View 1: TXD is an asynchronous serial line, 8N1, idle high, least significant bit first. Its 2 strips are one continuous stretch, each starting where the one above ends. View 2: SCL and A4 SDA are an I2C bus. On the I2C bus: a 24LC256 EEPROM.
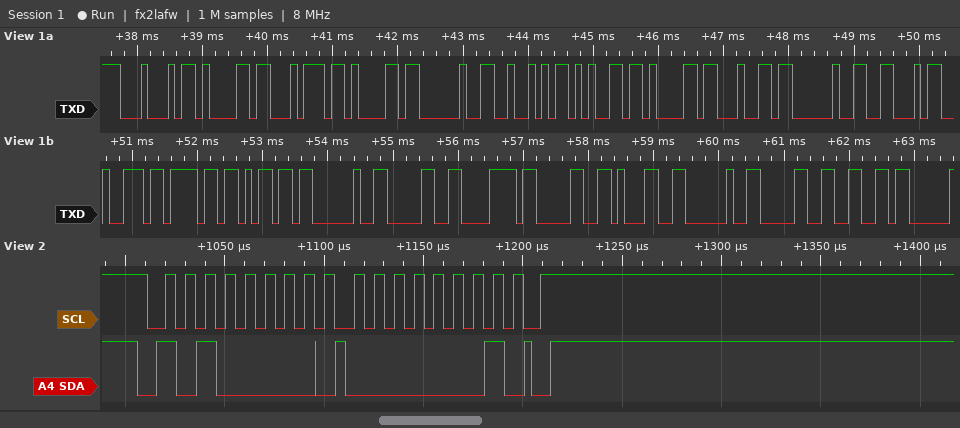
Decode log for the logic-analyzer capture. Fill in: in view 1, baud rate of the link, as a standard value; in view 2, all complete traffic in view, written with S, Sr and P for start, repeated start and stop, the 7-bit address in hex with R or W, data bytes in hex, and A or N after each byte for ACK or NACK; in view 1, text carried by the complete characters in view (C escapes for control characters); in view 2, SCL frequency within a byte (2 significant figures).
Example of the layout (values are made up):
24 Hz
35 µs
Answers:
9600 baud
S 50W A 01 A P
"Data Read From 0x01 0f"
100 kHz
